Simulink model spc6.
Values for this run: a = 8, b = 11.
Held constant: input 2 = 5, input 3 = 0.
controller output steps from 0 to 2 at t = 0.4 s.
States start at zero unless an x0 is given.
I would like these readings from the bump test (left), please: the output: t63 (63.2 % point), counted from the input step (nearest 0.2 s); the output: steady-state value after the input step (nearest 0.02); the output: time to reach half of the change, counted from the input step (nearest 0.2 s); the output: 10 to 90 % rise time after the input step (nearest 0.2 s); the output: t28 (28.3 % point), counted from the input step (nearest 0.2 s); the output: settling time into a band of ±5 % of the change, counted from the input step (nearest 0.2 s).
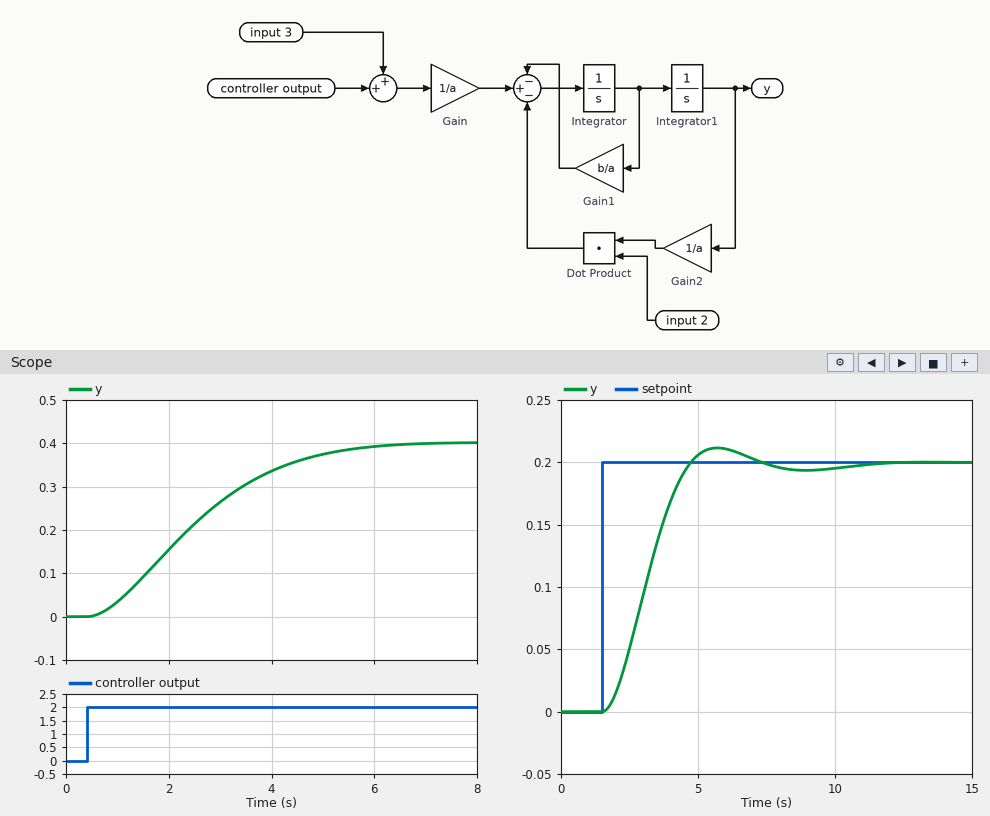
2.4 s
0.40
2.0 s
3.4 s
1.2 s
4.8 s
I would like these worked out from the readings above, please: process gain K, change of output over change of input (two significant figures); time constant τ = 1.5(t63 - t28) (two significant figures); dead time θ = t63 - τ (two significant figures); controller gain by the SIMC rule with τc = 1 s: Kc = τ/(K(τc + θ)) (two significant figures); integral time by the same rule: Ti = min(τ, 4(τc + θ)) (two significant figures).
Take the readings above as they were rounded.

0.20
1.8 s
0.60 s
5.6
1.8 s
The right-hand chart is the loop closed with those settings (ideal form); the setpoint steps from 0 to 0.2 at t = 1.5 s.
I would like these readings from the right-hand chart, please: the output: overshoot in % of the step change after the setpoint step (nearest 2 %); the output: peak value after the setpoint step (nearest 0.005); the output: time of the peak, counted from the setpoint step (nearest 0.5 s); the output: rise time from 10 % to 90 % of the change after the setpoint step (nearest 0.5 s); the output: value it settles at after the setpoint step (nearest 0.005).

6 %
0.210
4.0 s
2.0 s
0.200
